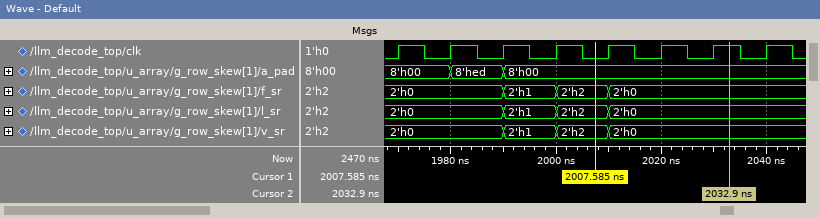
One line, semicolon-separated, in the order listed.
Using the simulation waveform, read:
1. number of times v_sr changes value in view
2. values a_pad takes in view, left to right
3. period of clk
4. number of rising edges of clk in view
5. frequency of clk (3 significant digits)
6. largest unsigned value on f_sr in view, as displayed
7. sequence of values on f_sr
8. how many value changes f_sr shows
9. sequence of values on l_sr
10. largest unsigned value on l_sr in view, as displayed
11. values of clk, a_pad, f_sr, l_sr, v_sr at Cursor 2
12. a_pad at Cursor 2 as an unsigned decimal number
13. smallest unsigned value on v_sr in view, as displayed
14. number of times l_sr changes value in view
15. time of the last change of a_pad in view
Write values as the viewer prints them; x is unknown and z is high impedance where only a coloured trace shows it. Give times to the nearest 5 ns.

3; 8'h00, 8'hed, 8'h00; 10 ns; 8; 100 MHz; 2'h2; 2'h0, 2'h1, 2'h2, 2'h0; 3; 2'h0, 2'h1, 2'h2, 2'h0; 2'h2; clk=1, a_pad=8'h00, f_sr=2'h0, l_sr=2'h0, v_sr=2'h0; 0; 2'h0; 3; 1990 ns
